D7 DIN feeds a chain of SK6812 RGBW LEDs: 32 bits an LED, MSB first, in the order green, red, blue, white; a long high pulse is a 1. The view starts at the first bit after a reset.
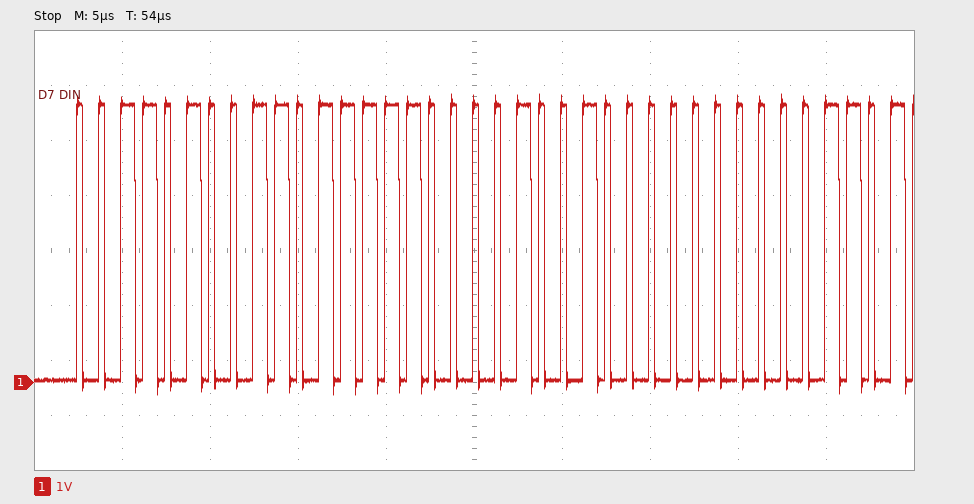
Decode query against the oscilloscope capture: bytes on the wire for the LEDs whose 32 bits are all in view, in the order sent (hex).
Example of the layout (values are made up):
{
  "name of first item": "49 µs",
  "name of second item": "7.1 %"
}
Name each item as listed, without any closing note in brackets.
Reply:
{
  "bytes on the wire for the LEDs whose 32 bits are all in view, in the order sent": "34 DF 09 00"
}
